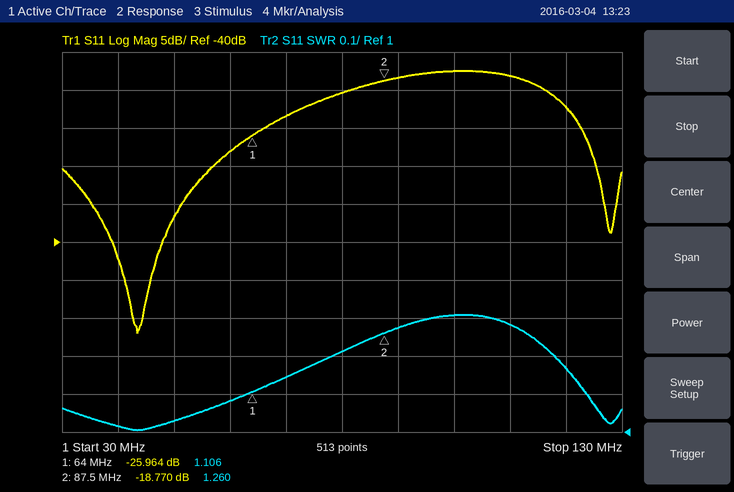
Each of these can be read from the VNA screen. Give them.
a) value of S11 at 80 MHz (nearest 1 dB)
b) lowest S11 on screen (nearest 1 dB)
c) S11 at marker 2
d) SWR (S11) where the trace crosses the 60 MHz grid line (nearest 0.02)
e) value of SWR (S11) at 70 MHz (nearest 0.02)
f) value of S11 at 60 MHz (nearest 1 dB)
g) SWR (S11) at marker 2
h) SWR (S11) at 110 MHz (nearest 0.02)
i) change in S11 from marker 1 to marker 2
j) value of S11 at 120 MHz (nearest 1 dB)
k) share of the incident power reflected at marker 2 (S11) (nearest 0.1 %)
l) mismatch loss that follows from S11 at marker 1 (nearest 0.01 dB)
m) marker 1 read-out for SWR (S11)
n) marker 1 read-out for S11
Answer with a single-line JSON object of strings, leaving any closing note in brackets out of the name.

{"value of S11 at 80 MHz": "-20 dB", "lowest S11 on screen": "-52 dB", "S11 at marker 2": "-18.770 dB", "SWR (S11) where the trace crosses the 60 MHz grid line": "1.08", "value of SWR (S11) at 70 MHz": "1.14", "value of S11 at 60 MHz": "-28 dB", "SWR (S11) at marker 2": "1.260", "SWR (S11) at 110 MHz": "1.28", "change in S11 from marker 1 to marker 2": "7.194 dB", "value of S11 at 120 MHz": "-22 dB", "share of the incident power reflected at marker 2 (S11)": "1.3 %", "mismatch loss that follows from S11 at marker 1": "0.01 dB", "marker 1 read-out for SWR": "1.106", "marker 1 read-out for S11": "-25.964 dB"}
